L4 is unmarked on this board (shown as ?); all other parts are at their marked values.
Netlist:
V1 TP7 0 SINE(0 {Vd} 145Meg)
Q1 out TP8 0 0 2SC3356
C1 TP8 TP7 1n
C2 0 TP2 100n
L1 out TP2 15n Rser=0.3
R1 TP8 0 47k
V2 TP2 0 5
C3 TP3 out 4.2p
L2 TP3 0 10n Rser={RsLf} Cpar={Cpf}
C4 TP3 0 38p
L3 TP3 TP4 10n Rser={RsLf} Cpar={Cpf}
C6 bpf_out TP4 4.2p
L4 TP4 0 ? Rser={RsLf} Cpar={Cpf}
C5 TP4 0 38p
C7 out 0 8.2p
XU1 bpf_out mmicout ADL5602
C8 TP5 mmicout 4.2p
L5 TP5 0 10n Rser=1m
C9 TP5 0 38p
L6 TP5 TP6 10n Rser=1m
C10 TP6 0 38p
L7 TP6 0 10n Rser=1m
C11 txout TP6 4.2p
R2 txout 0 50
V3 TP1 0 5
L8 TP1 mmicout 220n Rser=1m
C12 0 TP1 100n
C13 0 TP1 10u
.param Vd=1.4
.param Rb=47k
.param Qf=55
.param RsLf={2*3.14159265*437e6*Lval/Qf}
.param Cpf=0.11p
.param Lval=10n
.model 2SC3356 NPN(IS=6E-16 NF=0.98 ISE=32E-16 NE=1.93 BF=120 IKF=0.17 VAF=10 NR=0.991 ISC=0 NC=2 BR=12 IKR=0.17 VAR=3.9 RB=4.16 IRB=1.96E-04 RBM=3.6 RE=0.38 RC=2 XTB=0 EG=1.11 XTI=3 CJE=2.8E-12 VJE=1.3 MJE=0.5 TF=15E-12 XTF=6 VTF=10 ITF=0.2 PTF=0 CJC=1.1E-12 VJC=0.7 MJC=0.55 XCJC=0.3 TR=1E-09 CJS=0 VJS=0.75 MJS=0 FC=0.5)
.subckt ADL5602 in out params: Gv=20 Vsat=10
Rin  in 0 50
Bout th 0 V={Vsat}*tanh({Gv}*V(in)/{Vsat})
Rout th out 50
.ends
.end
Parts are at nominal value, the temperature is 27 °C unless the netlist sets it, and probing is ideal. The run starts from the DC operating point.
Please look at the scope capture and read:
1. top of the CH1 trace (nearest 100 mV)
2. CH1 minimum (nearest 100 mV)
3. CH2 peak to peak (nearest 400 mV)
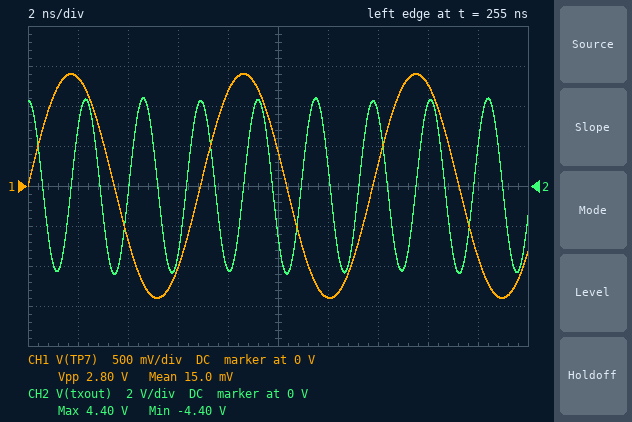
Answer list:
1.4 V
-1.4 V
8.8 V
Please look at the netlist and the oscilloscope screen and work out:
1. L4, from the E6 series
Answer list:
22 nH
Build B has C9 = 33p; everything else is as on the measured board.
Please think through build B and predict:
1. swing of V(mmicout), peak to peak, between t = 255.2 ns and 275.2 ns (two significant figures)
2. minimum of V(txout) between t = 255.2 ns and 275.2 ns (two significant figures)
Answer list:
11 V
-4.2 V
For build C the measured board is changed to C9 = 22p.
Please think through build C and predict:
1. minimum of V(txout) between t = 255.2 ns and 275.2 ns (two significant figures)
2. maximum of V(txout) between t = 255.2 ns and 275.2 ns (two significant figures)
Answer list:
-1.4 V
1.4 V
